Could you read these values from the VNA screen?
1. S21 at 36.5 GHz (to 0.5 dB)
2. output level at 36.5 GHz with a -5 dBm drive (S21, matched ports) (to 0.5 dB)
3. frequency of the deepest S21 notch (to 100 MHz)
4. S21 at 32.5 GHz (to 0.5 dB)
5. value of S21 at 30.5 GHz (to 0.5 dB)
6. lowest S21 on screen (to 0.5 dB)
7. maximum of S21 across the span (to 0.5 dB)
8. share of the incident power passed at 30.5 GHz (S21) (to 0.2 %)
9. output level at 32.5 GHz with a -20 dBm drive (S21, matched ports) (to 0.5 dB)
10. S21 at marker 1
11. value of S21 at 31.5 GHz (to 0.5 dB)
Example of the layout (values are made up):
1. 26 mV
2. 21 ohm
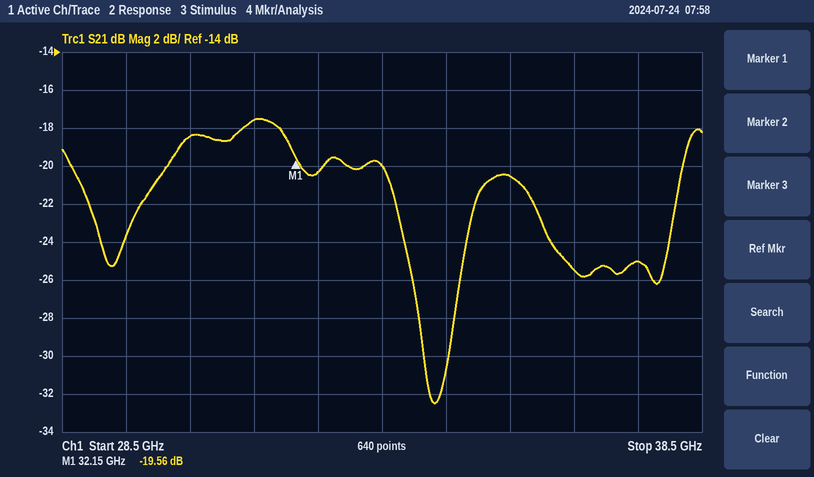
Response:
1. -25.5 dB
2. -30.5 dBm
3. 34.3 GHz
4. -20.5 dB
5. -18.5 dB
6. -32.5 dB
7. -17.5 dB
8. 1.4 %
9. -40.5 dBm
10. -19.56 dB
11. -17.5 dB
